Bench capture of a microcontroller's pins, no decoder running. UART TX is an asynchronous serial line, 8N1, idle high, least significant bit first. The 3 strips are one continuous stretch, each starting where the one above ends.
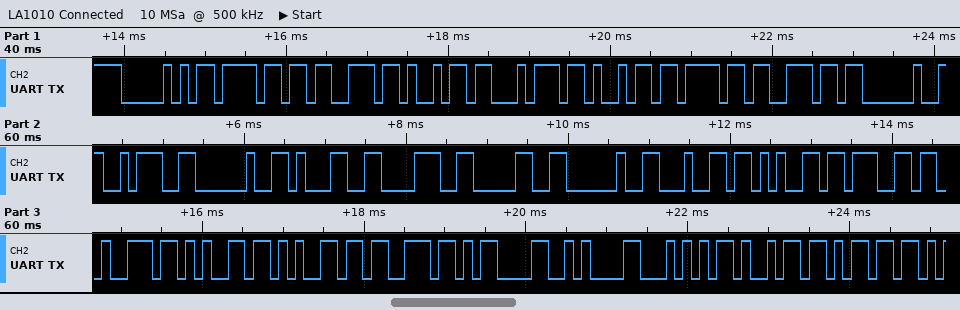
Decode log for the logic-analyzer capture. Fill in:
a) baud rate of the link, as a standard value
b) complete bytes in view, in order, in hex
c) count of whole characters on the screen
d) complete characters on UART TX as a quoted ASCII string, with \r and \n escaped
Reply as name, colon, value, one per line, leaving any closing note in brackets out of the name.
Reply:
baud rate of the link, as a standard value: 9600 baud
complete bytes in view, in order, in hex: 50 6F 73 69 74 69 6F 6E 20 3A 20 31 38 30 20 64 65 67 72 65 65 73 0D 0A 54 69 6D
count of whole characters on the screen: 27
complete characters on UART TX as a quoted ASCII string, with \r and \n escaped: "Position : 180 degrees\r\nTim"
